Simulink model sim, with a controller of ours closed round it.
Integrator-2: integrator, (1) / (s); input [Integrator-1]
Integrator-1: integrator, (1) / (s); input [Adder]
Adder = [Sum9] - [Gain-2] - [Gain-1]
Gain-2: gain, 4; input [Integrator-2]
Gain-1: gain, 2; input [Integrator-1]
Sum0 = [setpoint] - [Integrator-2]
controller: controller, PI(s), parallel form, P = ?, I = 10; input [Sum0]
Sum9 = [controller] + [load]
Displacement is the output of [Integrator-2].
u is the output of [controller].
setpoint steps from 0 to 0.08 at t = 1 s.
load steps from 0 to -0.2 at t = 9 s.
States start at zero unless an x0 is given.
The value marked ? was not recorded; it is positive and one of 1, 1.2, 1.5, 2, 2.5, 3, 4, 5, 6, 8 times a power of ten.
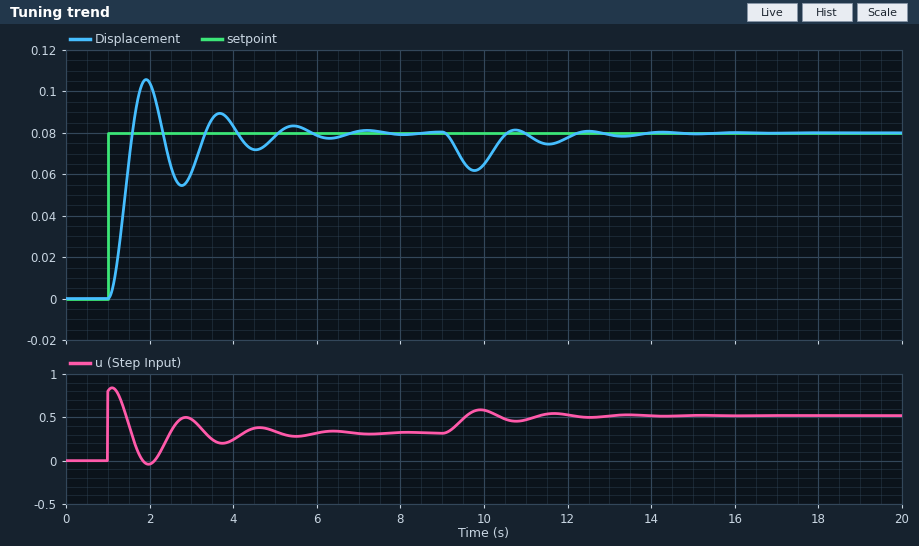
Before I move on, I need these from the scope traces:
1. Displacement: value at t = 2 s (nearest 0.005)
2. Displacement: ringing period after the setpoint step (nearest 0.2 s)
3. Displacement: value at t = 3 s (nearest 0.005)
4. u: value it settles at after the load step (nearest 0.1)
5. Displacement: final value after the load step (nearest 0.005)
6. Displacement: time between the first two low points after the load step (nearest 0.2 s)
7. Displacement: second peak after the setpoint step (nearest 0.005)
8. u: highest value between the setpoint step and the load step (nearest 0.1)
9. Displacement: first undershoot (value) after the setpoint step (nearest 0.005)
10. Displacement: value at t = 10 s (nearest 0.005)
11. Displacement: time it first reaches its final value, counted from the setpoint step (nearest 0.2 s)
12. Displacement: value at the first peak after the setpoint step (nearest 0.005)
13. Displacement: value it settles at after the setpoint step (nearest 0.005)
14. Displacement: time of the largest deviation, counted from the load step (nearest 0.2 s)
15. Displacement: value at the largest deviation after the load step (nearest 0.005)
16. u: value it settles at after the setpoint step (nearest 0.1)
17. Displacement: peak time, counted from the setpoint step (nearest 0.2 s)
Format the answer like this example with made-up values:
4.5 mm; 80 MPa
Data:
0.105; 1.8 s; 0.060; 0.5; 0.080; 1.8 s; 0.090; 0.8; 0.055; 0.065; 0.6 s; 0.105; 0.080; 0.8 s; 0.060; 0.3; 1.0 s
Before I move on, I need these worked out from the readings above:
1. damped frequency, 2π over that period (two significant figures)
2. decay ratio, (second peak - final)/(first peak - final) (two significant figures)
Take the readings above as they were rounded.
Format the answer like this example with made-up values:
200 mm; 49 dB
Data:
3.5 rad/s; 0.40
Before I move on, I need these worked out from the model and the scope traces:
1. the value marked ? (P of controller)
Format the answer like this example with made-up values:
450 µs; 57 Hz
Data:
10
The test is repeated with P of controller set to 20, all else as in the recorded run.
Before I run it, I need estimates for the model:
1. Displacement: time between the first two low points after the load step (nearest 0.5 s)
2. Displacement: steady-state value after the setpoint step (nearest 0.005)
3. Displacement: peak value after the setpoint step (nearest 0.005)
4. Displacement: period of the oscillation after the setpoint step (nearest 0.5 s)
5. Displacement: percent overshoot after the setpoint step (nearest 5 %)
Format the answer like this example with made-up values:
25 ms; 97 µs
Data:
1.5 s; 0.080; 0.110; 1.5 s; 40 %
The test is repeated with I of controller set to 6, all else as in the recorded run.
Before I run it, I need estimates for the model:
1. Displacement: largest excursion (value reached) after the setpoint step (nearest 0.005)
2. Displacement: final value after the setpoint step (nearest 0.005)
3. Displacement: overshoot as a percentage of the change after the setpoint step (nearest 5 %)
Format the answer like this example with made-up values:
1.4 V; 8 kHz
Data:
0.095; 0.080; 20 %
